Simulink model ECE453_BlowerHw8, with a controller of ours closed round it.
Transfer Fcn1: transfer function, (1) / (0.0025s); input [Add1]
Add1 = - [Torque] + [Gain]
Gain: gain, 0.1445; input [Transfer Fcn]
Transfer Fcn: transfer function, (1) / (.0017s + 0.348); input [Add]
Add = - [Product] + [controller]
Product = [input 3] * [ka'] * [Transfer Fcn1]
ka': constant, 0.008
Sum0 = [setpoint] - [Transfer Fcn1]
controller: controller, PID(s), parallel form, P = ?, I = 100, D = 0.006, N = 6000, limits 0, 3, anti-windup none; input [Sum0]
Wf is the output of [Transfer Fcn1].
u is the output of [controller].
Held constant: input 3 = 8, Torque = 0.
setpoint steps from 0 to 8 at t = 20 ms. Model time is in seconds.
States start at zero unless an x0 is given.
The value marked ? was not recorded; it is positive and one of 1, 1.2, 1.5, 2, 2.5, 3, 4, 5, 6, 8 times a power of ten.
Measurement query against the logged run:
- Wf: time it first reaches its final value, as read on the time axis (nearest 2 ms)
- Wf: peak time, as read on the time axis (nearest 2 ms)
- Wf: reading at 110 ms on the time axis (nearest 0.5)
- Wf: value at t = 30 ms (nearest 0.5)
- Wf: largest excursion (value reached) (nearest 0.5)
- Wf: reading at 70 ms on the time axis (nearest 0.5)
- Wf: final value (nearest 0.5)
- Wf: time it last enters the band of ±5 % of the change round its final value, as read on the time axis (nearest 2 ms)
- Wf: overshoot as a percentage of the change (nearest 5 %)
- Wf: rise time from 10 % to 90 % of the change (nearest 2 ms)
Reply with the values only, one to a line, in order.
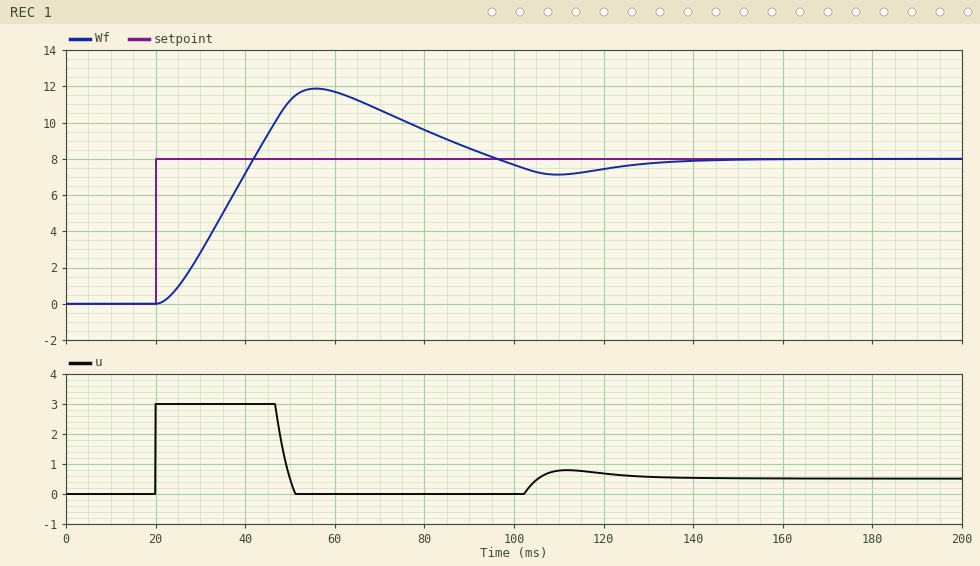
42 ms
56 ms
7.0
3.0
12.0
10.5
8.0
124 ms
50 %
16 ms
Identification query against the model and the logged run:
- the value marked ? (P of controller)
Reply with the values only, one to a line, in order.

2
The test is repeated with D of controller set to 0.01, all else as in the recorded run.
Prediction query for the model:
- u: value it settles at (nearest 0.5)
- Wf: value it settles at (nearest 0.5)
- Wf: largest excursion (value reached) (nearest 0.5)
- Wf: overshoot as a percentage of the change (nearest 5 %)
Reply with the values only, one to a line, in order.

0.5
8.0
11.5
45 %
